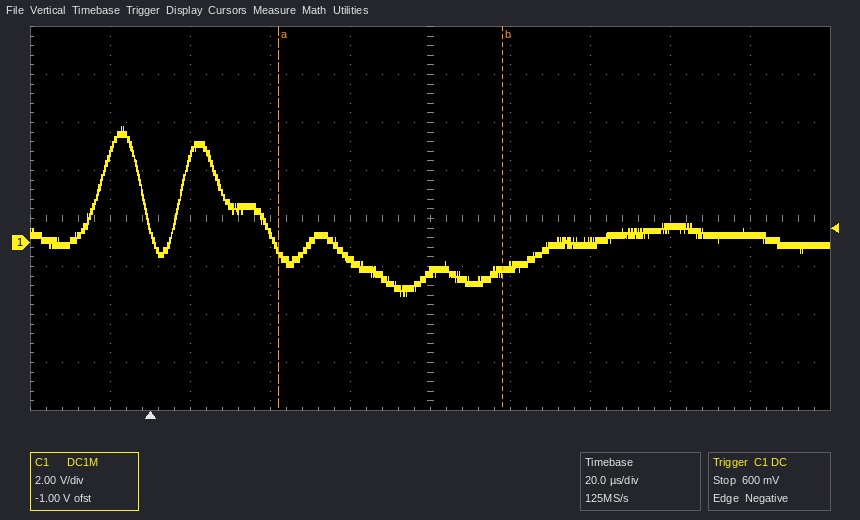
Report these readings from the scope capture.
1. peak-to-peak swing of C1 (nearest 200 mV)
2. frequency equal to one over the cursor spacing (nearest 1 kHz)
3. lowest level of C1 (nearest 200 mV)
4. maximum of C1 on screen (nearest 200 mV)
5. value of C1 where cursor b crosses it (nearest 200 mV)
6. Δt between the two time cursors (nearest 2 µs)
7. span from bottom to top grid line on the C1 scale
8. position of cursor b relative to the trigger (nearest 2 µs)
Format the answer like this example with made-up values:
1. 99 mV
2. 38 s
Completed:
1. 7.0 V
2. 18 kHz
3. -2.2 V
4. 4.8 V
5. -1.2 V
6. 56 µs
7. 16 V
8. +88 µs
